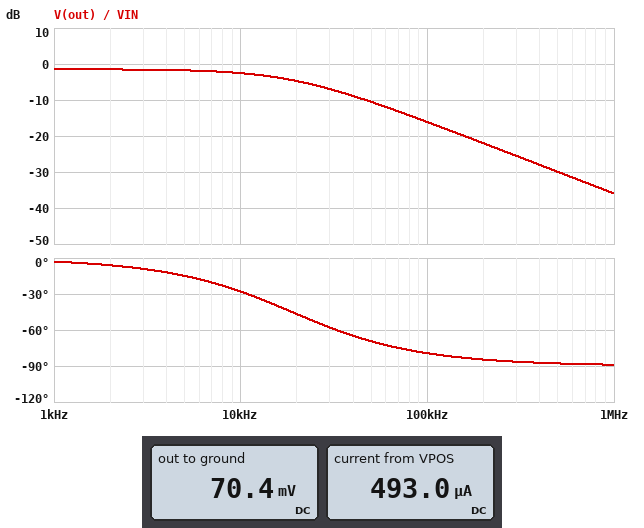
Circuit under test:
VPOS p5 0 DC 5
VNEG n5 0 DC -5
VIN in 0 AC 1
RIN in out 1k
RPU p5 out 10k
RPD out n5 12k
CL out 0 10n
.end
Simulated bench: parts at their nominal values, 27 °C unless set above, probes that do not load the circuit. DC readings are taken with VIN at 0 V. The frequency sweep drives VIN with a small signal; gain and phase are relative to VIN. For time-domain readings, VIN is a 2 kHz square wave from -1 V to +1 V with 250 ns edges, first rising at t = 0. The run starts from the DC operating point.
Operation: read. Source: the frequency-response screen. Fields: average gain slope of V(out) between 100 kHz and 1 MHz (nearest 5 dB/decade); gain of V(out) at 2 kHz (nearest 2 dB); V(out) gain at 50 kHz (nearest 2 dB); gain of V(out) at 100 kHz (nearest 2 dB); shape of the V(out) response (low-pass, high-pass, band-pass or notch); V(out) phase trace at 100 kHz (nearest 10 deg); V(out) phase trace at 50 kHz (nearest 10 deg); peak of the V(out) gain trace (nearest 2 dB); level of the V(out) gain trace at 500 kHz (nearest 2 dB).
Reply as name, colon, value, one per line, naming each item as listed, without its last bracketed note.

average gain slope of V(out) between 100 kHz and 1 MHz: -20 dB/decade
gain of V(out) at 2 kHz: -2 dB
V(out) gain at 50 kHz: -10 dB
gain of V(out) at 100 kHz: -16 dB
shape of the V(out) response: low-pass
V(out) phase trace at 100 kHz: -80 deg
V(out) phase trace at 50 kHz: -70 deg
peak of the V(out) gain trace: -2 dB
level of the V(out) gain trace at 500 kHz: -30 dB
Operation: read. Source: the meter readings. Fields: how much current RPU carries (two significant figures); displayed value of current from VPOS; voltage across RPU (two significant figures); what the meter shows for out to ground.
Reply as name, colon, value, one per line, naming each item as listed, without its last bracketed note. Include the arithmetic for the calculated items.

how much current RPU carries: (5 V - 70.4 mV) / 10 kΩ = 490 µA
displayed value of current from VPOS: 493.0 µA
voltage across RPU: 5 V - 70.4 mV = 4.9 V
what the meter shows for out to ground: 70.4 mV
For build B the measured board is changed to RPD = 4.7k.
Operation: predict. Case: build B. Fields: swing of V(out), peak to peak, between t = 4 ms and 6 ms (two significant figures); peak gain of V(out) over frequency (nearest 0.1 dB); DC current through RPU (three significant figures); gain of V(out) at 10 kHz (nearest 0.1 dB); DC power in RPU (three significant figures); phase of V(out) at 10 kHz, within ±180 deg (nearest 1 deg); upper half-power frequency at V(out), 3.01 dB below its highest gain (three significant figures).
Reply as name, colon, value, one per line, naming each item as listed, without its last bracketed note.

swing of V(out), peak to peak, between t = 4 ms and 6 ms: 1.5 V
peak gain of V(out) over frequency: -2.4 dB
DC current through RPU: 543 µA
gain of V(out) at 10 kHz: -3.3 dB
DC power in RPU: 2.95 mW
phase of V(out) at 10 kHz, within ±180 deg: -26 deg
upper half-power frequency at V(out), 3.01 dB below its highest gain: 20.9 kHz
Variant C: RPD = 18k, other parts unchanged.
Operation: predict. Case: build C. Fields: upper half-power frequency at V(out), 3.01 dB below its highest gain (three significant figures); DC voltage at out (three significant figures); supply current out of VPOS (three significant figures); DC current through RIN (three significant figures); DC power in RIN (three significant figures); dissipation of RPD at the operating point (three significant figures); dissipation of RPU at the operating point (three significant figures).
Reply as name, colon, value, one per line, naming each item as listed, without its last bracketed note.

upper half-power frequency at V(out), 3.01 dB below its highest gain: 18.4 kHz
DC voltage at out: 192 mV
supply current out of VPOS: 481 µA
DC current through RIN: 192 µA
DC power in RIN: 37.0 µW
dissipation of RPD at the operating point: 1.50 mW
dissipation of RPU at the operating point: 2.31 mW
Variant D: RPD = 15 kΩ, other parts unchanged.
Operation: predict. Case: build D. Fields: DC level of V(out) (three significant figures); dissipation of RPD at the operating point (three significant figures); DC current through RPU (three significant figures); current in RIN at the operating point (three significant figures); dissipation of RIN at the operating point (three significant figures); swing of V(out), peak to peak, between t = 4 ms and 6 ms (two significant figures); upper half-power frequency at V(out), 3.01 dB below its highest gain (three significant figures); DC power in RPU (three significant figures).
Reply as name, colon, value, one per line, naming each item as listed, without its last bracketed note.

DC level of V(out): 143 mV
dissipation of RPD at the operating point: 1.76 mW
DC current through RPU: 486 µA
current in RIN at the operating point: 143 µA
dissipation of RIN at the operating point: 20.4 µW
swing of V(out), peak to peak, between t = 4 ms and 6 ms: 1.7 V
upper half-power frequency at V(out), 3.01 dB below its highest gain: 18.6 kHz
DC power in RPU: 2.36 mW
